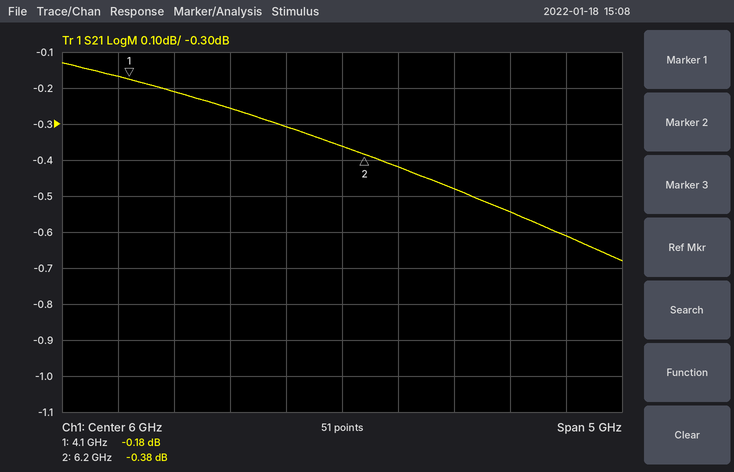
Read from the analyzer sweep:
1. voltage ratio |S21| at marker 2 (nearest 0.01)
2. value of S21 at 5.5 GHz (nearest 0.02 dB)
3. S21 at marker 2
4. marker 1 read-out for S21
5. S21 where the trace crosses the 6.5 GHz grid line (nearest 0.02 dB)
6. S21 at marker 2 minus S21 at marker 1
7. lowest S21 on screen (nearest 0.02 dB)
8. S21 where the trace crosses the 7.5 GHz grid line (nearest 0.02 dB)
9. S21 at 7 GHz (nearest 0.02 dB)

0.96
-0.30 dB
-0.38 dB
-0.18 dB
-0.42 dB
-0.20 dB
-0.68 dB
-0.54 dB
-0.48 dB
